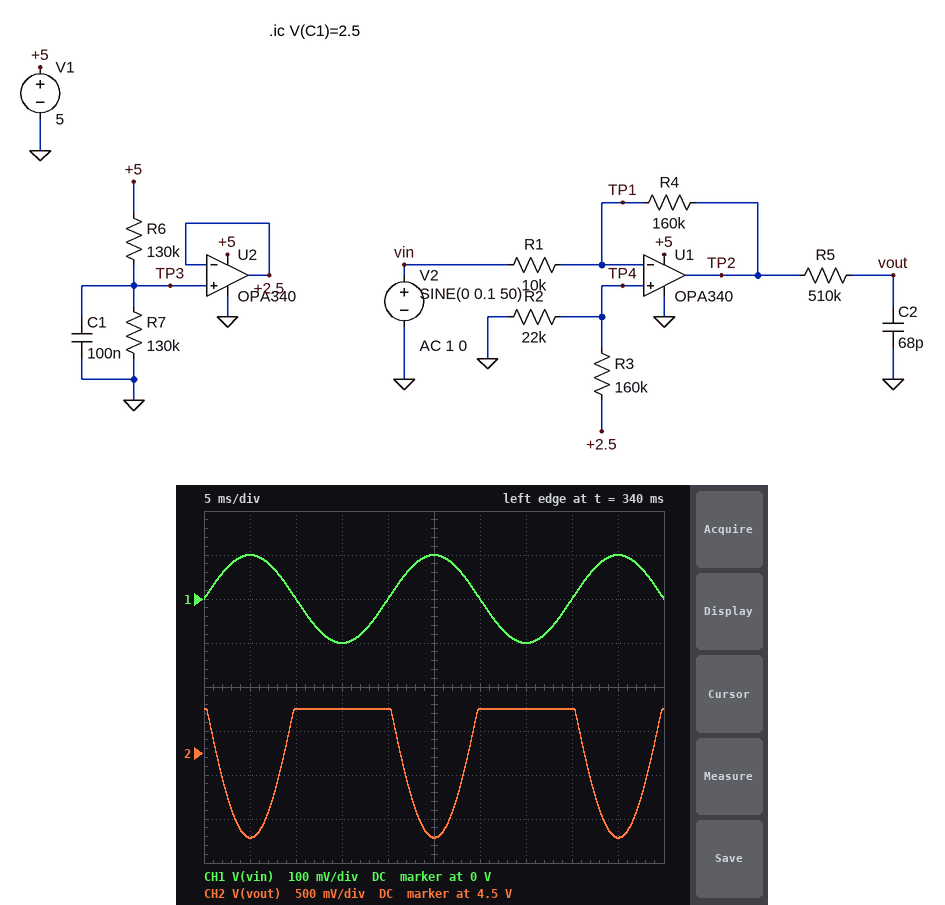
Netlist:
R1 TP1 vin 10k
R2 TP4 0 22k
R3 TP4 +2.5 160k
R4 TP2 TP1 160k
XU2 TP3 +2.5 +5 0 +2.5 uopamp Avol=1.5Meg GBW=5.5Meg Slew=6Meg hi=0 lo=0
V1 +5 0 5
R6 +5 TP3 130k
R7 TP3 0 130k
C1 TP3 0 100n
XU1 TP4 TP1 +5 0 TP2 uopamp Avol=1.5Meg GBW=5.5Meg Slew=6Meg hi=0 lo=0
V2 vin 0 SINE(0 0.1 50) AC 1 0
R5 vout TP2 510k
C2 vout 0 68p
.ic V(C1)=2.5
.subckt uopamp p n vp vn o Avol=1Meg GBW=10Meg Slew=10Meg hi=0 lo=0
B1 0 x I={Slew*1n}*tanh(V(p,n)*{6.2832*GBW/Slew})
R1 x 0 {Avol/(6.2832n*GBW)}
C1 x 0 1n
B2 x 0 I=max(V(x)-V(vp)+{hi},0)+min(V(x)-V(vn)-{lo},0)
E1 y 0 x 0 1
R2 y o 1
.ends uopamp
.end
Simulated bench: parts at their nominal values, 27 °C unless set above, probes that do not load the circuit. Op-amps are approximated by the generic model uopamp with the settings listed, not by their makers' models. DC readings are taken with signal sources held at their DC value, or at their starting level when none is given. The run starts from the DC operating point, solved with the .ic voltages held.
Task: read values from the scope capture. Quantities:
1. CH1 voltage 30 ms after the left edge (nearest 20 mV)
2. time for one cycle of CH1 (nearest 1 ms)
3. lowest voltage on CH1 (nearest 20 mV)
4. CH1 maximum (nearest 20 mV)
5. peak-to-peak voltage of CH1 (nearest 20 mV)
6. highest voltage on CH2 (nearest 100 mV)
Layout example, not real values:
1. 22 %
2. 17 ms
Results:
1. 0 V
2. 20 ms
3. -100 mV
4. 100 mV
5. 200 mV
6. 5.0 V
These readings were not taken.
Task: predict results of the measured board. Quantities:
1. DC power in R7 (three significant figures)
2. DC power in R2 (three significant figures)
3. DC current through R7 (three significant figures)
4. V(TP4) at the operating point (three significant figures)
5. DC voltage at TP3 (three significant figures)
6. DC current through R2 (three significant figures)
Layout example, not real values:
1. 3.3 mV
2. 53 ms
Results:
1. 48.1 µW
2. 4.15 µW
3. 19.2 µA
4. 302 mV
5. 2.50 V
6. 13.7 µA
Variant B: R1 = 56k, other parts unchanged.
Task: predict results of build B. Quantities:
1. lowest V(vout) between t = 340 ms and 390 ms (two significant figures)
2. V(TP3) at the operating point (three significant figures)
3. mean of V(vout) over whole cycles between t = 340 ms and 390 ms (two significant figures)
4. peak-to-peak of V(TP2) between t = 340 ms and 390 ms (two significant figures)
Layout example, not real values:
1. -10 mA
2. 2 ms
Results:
1. 880 mV
2. 2.50 V
3. 1.2 V
4. 570 mV
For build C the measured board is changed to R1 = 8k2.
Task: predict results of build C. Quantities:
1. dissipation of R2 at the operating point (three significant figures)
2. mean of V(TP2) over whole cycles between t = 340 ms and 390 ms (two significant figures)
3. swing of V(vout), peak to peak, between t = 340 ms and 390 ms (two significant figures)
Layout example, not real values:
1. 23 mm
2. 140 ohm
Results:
1. 4.15 µW
2. 4.9 V
3. 760 mV
